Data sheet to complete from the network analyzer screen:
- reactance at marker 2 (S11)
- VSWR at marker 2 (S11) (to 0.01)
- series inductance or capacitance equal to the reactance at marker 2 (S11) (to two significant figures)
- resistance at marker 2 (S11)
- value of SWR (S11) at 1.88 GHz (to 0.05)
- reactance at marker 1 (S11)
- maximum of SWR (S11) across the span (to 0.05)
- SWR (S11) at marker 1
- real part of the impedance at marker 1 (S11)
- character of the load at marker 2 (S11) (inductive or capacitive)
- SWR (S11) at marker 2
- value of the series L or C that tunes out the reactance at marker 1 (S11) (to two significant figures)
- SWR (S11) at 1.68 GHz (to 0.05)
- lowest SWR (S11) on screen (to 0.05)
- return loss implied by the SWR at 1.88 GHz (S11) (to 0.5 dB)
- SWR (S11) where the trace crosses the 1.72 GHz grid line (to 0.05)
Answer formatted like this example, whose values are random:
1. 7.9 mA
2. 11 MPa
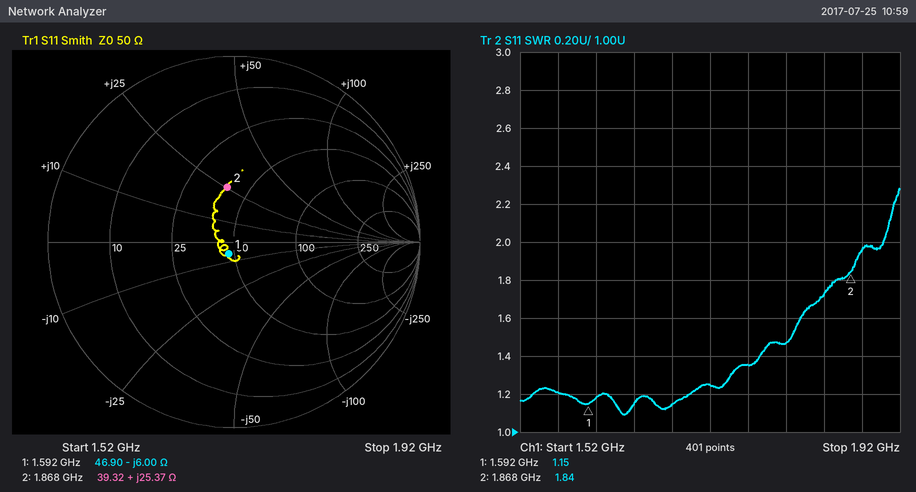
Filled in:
1. +25.37 Ω
2. 1.84
3. 2.2 nH
4. 39.32 Ω
5. 1.95
6. -6.00 Ω
7. 2.30
8. 1.15
9. 46.90 Ω
10. inductive
11. 1.84
12. 600 pH
13. 1.15
14. 1.10
15. 10.0 dB
16. 1.25
